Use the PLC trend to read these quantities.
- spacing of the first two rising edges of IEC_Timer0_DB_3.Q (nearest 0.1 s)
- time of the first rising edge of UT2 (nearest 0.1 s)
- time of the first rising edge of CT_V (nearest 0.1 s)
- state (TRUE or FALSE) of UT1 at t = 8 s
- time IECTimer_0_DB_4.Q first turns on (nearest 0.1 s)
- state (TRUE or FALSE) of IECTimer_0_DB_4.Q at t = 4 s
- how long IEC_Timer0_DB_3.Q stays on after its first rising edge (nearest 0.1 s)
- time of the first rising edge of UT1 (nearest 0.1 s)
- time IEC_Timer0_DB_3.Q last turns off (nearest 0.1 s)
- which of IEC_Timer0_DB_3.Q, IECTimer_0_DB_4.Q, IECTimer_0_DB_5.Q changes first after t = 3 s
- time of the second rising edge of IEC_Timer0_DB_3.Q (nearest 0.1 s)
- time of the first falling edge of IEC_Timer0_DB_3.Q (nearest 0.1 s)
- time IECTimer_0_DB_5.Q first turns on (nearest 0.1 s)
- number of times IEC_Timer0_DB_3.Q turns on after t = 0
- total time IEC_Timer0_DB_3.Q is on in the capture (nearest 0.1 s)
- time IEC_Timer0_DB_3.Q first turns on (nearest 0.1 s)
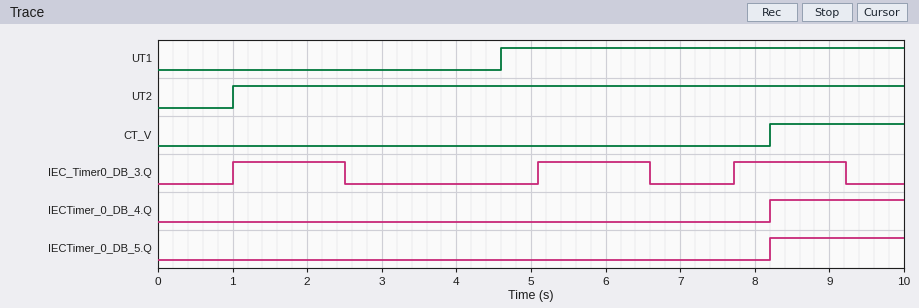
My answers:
4.1 s
1.0 s
8.2 s
TRUE
8.2 s
FALSE
1.5 s
4.6 s
9.2 s
IEC_Timer0_DB_3.Q
5.1 s
2.5 s
8.2 s
3
4.5 s
1.0 s
